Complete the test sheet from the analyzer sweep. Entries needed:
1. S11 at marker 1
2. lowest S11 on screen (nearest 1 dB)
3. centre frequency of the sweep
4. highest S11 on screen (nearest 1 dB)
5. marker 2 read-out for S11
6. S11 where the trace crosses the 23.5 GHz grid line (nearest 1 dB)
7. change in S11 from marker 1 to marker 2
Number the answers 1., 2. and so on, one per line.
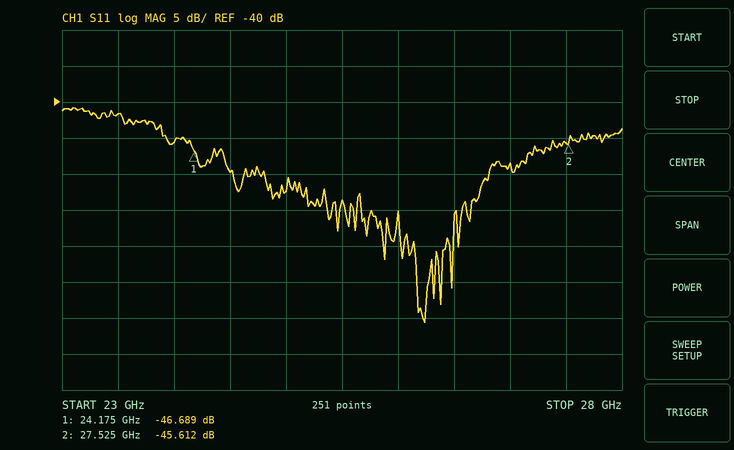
1. -46.689 dB
2. -71 dB
3. 25.5 GHz
4. -41 dB
5. -45.612 dB
6. -42 dB
7. 1.077 dB
